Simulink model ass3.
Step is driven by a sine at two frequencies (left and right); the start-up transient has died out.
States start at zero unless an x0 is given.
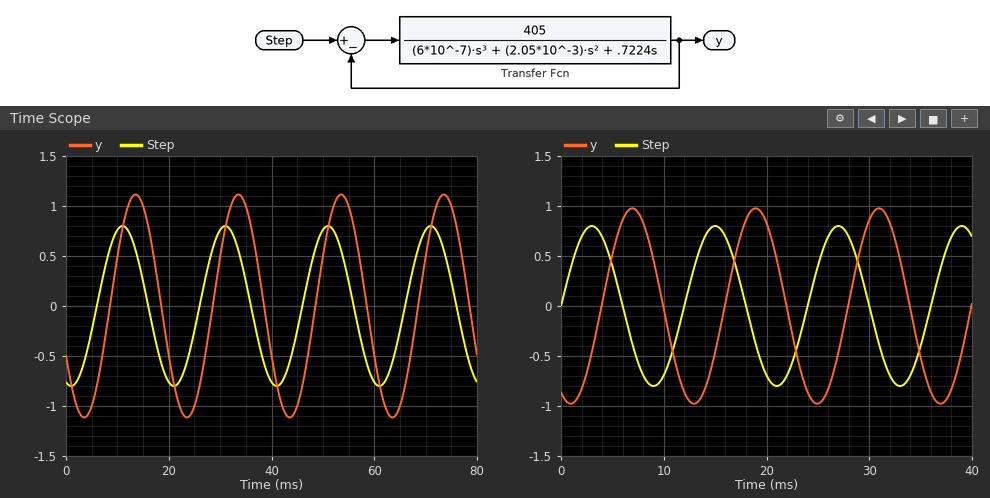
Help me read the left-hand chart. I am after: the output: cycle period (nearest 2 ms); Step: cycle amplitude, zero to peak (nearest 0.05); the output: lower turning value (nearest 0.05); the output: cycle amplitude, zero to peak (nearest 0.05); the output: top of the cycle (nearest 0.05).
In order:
20 ms
0.80
-1.10
1.10
1.10
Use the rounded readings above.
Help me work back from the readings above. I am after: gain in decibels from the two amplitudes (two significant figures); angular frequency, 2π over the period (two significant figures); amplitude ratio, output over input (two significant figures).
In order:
2.8 dB
0.31 rad/ms
1.4
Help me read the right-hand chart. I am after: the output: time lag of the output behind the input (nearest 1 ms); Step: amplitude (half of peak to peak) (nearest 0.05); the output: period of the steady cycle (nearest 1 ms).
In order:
4 ms
0.80
12 ms
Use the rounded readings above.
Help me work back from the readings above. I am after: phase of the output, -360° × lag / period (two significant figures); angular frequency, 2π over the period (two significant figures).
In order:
-120°
0.52 rad/ms
